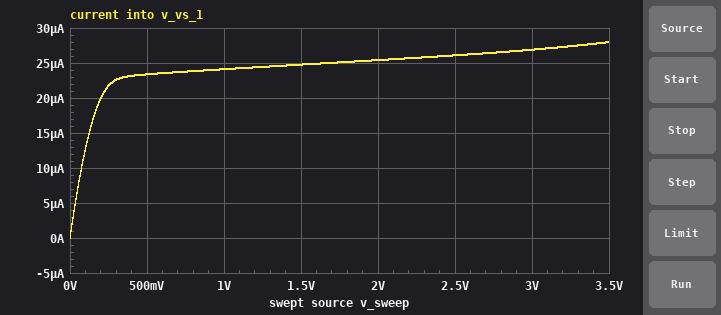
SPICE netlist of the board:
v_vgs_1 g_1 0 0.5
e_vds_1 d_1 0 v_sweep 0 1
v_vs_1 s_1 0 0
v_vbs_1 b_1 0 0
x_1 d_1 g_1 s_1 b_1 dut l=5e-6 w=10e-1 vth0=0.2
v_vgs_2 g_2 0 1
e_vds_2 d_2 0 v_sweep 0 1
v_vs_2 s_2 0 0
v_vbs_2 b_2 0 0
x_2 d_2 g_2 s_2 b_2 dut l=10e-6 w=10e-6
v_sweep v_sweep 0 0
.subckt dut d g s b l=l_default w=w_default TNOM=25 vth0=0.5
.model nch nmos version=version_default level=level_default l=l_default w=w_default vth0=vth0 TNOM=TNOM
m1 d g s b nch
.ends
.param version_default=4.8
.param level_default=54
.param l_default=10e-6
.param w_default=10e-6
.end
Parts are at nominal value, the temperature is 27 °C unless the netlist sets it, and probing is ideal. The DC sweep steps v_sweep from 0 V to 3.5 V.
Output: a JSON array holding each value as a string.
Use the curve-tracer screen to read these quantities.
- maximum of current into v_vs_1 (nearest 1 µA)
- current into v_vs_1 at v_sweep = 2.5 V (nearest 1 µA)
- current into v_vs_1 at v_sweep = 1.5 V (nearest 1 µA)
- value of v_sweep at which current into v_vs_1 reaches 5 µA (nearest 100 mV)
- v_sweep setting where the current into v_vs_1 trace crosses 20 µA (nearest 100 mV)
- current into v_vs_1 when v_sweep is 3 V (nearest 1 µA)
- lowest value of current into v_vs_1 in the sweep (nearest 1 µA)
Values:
["28 µA", "26 µA", "25 µA", "0 V", "200 mV", "27 µA", "0 A"]
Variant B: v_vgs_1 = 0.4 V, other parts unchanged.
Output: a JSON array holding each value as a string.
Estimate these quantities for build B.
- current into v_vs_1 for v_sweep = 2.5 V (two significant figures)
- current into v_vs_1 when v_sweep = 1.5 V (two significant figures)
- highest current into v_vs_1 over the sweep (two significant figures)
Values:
["12 µA", "11 µA", "13 µA"]
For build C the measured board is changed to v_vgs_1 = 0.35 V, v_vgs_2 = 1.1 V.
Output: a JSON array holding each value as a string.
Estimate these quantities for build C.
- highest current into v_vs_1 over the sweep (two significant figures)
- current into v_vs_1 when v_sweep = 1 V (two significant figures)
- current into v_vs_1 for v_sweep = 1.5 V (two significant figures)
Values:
["7.7 µA", "6.1 µA", "6.4 µA"]
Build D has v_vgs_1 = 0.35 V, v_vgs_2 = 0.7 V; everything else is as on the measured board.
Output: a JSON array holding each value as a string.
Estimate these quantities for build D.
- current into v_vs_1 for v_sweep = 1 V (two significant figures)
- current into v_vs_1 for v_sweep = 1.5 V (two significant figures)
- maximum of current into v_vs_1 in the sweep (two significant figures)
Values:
["6.1 µA", "6.4 µA", "7.7 µA"]
